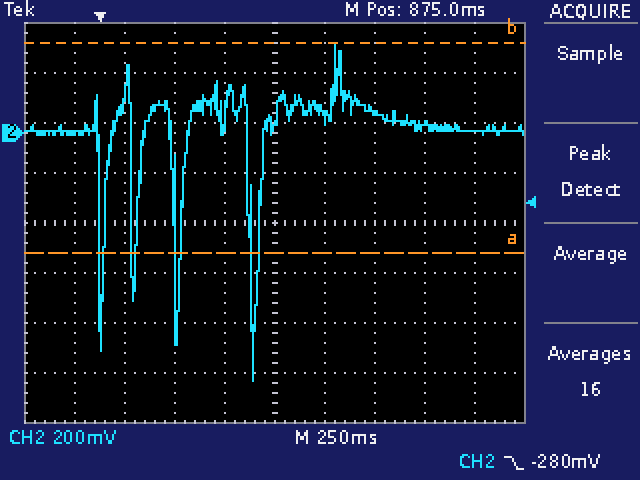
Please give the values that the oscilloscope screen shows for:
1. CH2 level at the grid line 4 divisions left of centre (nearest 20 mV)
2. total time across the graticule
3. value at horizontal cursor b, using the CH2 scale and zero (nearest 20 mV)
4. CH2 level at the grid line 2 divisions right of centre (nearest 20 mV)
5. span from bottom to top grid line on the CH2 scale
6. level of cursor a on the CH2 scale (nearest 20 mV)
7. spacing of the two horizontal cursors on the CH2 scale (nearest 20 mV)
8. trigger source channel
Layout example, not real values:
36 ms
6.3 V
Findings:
0 mV
2.5 s
360 mV
80 mV
1.6 V
-480 mV
840 mV
CH2
